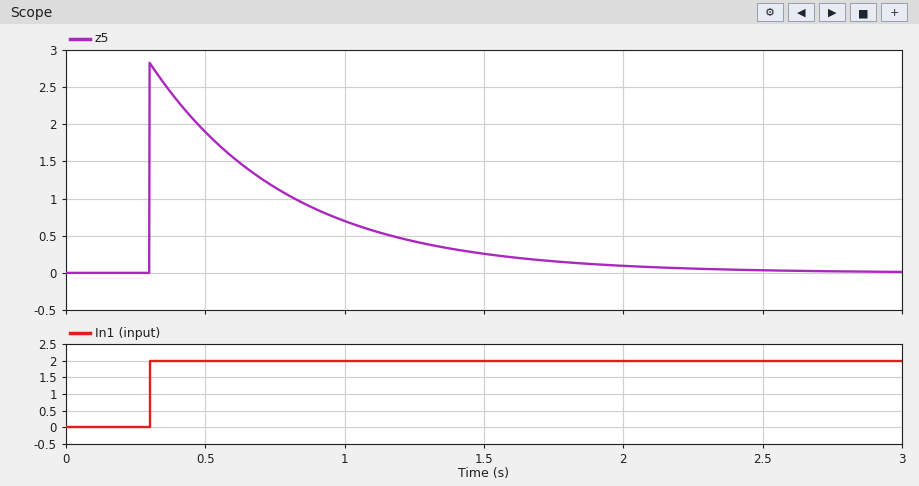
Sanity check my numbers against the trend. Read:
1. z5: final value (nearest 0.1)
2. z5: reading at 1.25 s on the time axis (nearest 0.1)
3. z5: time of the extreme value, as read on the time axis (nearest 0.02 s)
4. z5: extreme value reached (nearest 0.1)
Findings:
0.0
0.4
0.30 s
2.8
